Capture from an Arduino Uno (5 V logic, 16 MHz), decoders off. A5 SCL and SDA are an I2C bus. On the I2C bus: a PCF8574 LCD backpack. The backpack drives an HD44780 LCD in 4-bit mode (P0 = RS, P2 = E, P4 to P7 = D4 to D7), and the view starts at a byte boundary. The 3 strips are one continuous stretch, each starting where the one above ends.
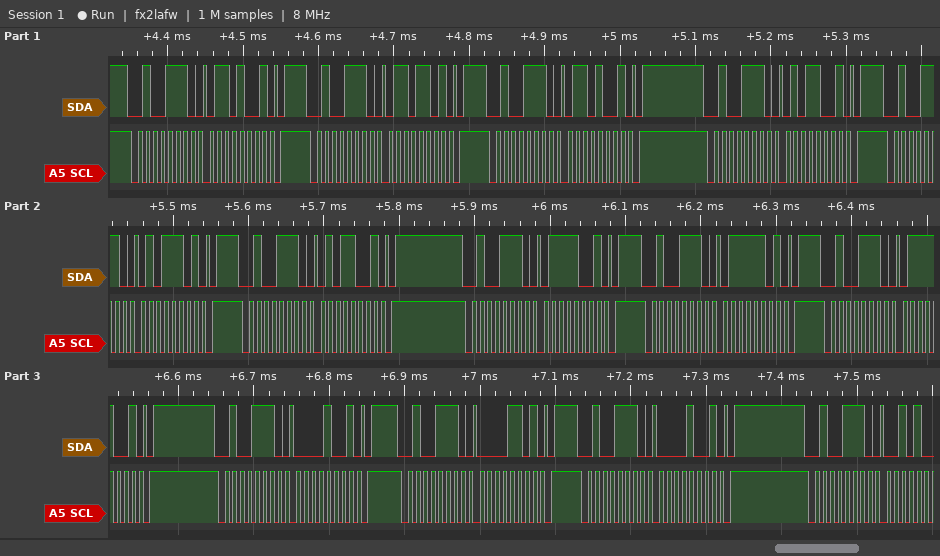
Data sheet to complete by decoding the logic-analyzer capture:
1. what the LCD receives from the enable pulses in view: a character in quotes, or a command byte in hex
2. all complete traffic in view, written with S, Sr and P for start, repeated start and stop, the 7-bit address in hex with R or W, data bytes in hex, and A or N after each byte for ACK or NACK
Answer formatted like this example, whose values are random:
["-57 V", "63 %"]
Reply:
["'e' 'p'", "S 27W A 69 A P S 27W A 6D A P S 27W A 69 A P S 27W A 59 A P S 27W A 5D A P S 27W A 59 A P S 27W A 79 A P S 27W A 7D A P S 27W A 79 A P S 27W A 09 A P S 27W A 0D A P S 27W A 09 A P S 27W A"]
